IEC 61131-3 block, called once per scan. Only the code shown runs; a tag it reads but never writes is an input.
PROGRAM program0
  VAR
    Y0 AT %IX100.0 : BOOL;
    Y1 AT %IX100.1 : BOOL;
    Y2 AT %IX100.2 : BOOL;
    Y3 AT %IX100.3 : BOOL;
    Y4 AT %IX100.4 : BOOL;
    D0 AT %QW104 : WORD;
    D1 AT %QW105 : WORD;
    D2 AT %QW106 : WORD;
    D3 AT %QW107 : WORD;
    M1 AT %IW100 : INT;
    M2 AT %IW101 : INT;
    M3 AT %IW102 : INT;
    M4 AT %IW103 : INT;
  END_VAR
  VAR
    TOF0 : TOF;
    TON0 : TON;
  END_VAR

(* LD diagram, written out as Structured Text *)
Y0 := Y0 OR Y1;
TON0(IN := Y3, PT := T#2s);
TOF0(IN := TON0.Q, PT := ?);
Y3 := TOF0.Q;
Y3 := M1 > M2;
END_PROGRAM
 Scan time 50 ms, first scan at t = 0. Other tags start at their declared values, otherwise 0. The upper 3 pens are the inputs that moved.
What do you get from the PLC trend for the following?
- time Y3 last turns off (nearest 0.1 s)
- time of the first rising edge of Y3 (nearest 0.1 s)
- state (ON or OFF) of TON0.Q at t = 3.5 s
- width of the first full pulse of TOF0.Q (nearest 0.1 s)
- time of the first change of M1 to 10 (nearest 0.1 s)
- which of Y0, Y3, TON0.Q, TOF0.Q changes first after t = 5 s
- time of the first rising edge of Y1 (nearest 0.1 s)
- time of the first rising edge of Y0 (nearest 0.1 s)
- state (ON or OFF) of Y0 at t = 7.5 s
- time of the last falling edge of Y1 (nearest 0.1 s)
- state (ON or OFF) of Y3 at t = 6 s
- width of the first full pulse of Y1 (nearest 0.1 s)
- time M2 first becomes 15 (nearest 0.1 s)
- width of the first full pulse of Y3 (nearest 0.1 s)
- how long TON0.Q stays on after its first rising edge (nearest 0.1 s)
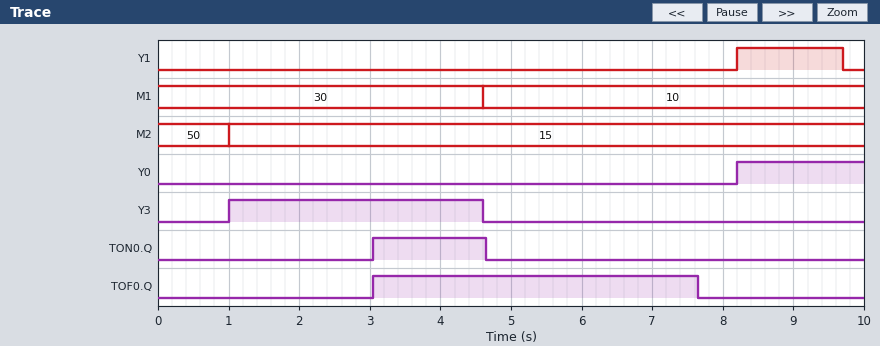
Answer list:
4.6 s
1.0 s
ON
4.6 s
4.6 s
TOF0.Q
8.2 s
8.2 s
OFF
9.7 s
OFF
1.5 s
1.0 s
3.6 s
1.6 s
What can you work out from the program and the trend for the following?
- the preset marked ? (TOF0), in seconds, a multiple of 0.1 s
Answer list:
3.0 s
